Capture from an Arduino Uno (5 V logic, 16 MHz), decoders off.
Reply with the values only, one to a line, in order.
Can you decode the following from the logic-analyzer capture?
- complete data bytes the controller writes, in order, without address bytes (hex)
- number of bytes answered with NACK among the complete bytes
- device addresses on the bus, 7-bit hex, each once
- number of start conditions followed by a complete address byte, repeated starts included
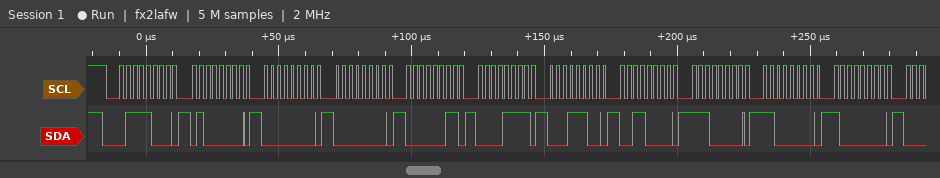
40 00 00 03 0F 1C 30 E0 C0 80
0
0x3C
1
